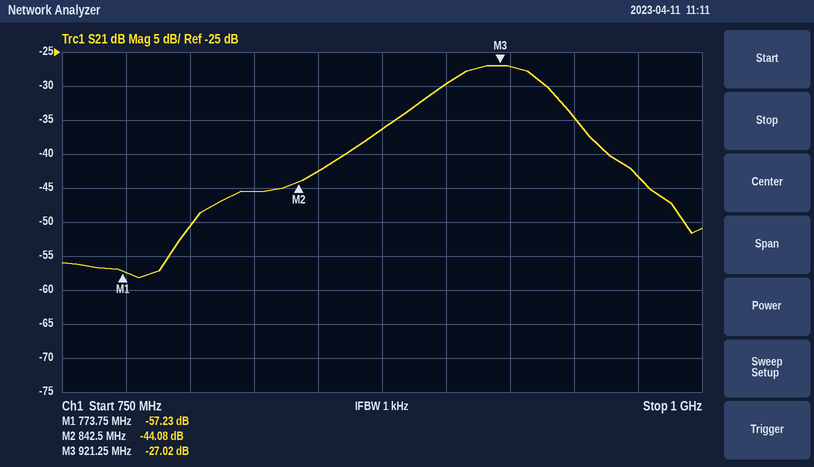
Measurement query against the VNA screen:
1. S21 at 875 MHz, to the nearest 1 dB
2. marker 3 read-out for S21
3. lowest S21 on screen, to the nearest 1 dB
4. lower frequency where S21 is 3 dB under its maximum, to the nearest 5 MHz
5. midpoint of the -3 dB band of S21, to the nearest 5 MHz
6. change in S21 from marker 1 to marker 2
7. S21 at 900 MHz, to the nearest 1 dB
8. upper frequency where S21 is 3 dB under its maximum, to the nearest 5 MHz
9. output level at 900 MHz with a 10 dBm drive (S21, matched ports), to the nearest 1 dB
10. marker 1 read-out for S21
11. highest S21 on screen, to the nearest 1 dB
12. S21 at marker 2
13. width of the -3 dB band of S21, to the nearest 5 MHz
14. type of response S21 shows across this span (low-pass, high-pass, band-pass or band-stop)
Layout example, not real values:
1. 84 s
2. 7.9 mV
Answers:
1. -36 dB
2. -27.02 dB
3. -58 dB
4. 900 MHz
5. 920 MHz
6. 13.15 dB
7. -30 dB
8. 940 MHz
9. -20 dBm
10. -57.23 dB
11. -27 dB
12. -44.08 dB
13. 40 MHz
14. band-pass
